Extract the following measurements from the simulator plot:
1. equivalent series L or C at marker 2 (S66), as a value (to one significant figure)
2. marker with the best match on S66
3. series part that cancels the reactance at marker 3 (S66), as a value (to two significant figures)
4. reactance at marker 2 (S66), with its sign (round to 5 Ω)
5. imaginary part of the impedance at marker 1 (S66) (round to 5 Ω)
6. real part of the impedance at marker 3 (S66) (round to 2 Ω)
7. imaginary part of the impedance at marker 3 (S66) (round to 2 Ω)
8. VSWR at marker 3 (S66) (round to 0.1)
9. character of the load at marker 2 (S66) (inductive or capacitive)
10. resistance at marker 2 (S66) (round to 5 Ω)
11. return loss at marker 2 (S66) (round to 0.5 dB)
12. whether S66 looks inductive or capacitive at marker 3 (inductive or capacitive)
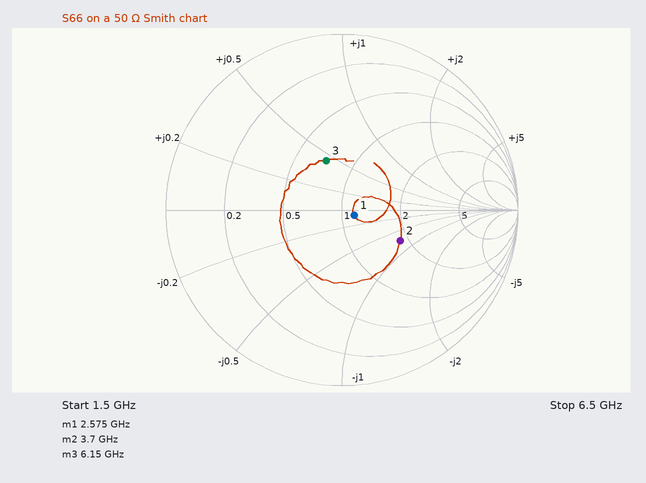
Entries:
1 pF
marker 1
1.2 pF
-35 Ω
-5 Ω
36 Ω
+22 Ω
1.8
capacitive
90 Ω
8.5 dB
inductive
